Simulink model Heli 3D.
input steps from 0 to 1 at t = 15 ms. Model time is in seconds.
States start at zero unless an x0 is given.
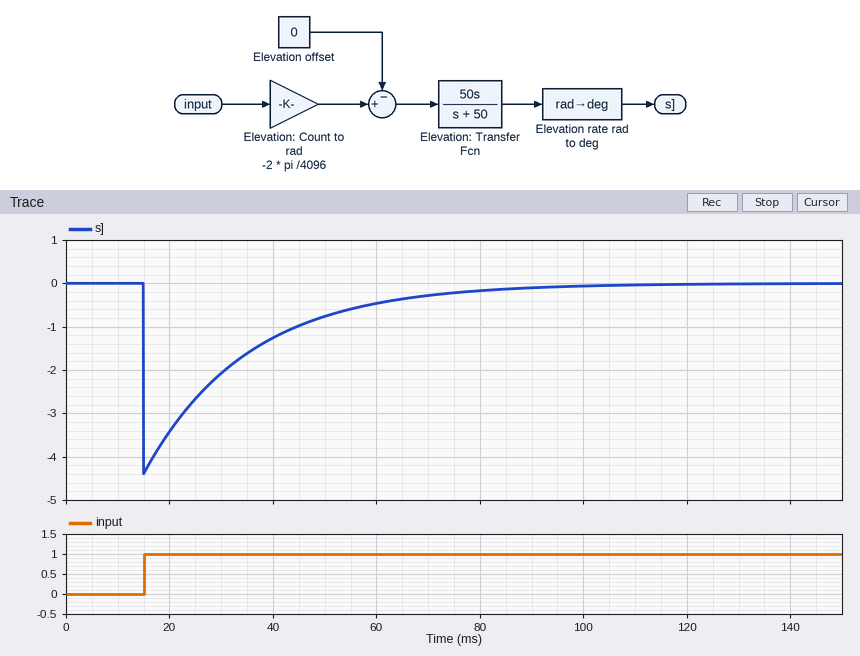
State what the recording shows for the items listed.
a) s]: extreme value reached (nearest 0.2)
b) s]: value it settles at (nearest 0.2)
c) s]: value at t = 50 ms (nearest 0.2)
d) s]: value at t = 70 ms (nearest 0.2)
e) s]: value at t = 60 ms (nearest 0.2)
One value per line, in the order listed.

-4.4
0.0
-0.8
-0.2
-0.4
